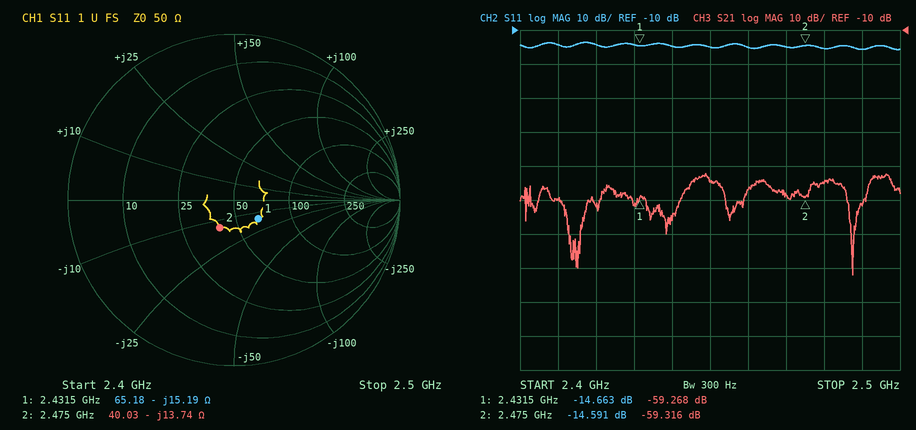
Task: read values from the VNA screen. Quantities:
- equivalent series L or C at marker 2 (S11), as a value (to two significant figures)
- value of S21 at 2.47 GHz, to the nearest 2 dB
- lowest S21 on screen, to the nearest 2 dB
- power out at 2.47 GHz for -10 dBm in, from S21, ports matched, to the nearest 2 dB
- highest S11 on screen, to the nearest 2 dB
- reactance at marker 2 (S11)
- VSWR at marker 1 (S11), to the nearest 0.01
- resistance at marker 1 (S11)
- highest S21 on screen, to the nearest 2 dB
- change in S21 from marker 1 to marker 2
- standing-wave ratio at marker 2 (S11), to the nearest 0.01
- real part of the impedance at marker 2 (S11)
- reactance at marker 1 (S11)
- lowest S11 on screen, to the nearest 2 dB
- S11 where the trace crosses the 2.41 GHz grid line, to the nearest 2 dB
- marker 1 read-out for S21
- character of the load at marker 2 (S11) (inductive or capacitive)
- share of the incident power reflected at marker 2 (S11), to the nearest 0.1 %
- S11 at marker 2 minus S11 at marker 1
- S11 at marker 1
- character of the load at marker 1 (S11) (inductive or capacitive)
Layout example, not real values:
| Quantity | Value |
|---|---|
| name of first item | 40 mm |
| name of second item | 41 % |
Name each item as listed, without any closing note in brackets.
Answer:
| Quantity | Value |
|---|---|
| equivalent series L or C at marker 2 (S11), as a value | 4.7 pF |
| value of S21 at 2.47 GHz, to the nearest 2 dB | -58 dB |
| lowest S21 on screen, to the nearest 2 dB | -82 dB |
| power out at 2.47 GHz for -10 dBm in, from S21, ports matched, to the nearest 2 dB | -68 dBm |
| highest S11 on screen, to the nearest 2 dB | -14 dB |
| reactance at marker 2 | -13.74 Ω |
| VSWR at marker 1 (S11), to the nearest 0.01 | 1.45 |
| resistance at marker 1 | 65.18 Ω |
| highest S21 on screen, to the nearest 2 dB | -52 dB |
| change in S21 from marker 1 to marker 2 | -0.048 dB |
| standing-wave ratio at marker 2 (S11), to the nearest 0.01 | 1.46 |
| real part of the impedance at marker 2 | 40.03 Ω |
| reactance at marker 1 | -15.19 Ω |
| lowest S11 on screen, to the nearest 2 dB | -16 dB |
| S11 where the trace crosses the 2.41 GHz grid line, to the nearest 2 dB | -14 dB |
| marker 1 read-out for S21 | -59.268 dB |
| character of the load at marker 2 (S11) | capacitive |
| share of the incident power reflected at marker 2 (S11), to the nearest 0.1 % | 3.5 % |
| S11 at marker 2 minus S11 at marker 1 | 0.072 dB |
| S11 at marker 1 | -14.663 dB |
| character of the load at marker 1 (S11) | capacitive |
